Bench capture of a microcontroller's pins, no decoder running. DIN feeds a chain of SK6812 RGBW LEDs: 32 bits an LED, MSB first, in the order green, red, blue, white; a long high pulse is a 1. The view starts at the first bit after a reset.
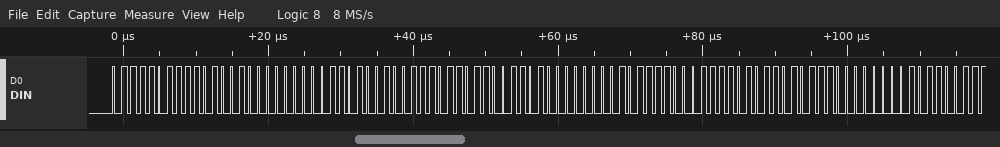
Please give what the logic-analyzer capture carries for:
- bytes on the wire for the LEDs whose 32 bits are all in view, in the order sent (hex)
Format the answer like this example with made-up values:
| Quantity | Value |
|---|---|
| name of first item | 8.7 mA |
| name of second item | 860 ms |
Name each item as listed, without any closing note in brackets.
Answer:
| Quantity | Value |
|---|---|
| bytes on the wire for the LEDs whose 32 bits are all in view, in the order sent | 7B D2 00 D2 76 CD 00 BC 7A D7 00 B3 |
